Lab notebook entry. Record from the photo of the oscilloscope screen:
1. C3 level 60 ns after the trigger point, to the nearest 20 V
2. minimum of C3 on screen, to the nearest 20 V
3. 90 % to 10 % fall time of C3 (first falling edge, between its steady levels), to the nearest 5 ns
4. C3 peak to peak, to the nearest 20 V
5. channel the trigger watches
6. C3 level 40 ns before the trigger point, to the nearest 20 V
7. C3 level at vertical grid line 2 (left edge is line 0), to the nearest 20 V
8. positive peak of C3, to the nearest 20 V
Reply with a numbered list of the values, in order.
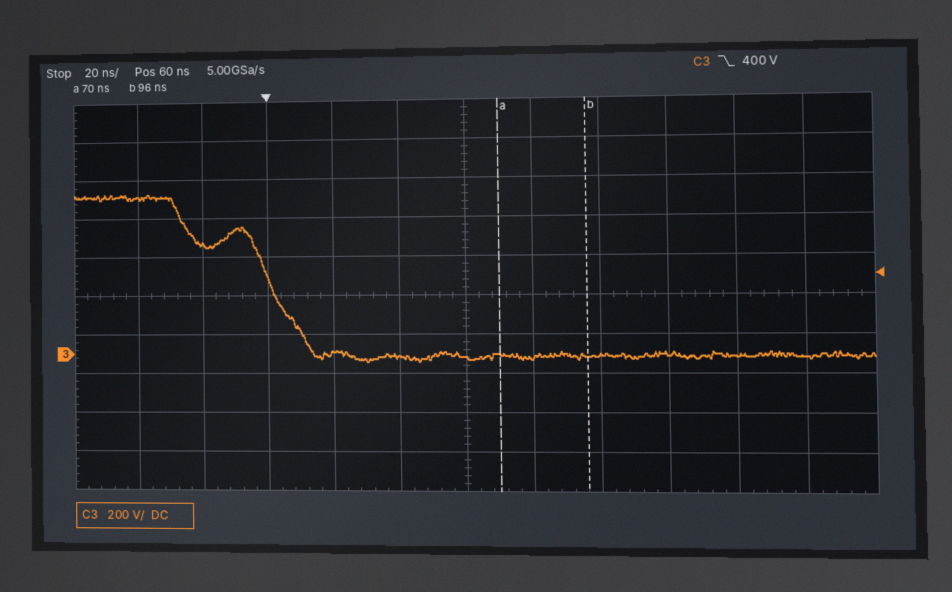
1. -20 V
2. -40 V
3. 40 ns
4. 860 V
5. C3
6. 800 V
7. 560 V
8. 820 V
